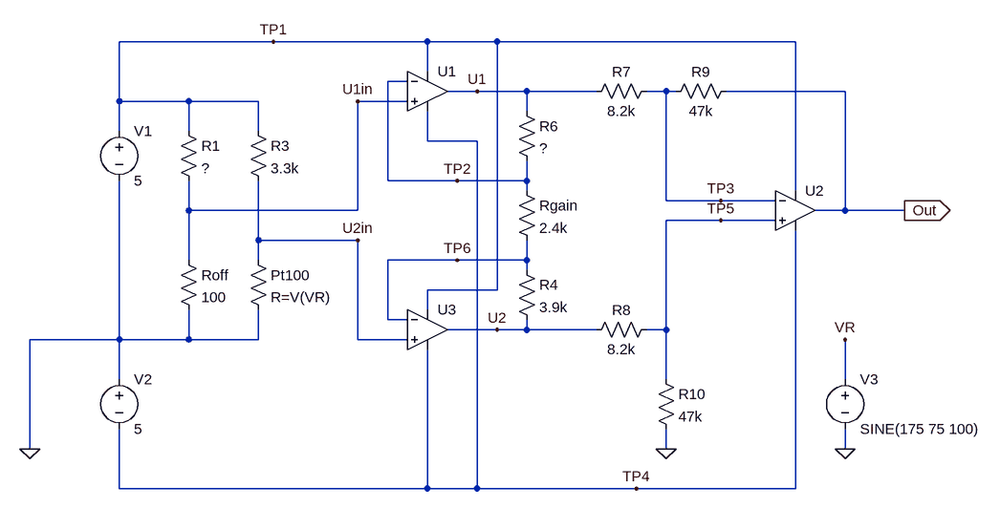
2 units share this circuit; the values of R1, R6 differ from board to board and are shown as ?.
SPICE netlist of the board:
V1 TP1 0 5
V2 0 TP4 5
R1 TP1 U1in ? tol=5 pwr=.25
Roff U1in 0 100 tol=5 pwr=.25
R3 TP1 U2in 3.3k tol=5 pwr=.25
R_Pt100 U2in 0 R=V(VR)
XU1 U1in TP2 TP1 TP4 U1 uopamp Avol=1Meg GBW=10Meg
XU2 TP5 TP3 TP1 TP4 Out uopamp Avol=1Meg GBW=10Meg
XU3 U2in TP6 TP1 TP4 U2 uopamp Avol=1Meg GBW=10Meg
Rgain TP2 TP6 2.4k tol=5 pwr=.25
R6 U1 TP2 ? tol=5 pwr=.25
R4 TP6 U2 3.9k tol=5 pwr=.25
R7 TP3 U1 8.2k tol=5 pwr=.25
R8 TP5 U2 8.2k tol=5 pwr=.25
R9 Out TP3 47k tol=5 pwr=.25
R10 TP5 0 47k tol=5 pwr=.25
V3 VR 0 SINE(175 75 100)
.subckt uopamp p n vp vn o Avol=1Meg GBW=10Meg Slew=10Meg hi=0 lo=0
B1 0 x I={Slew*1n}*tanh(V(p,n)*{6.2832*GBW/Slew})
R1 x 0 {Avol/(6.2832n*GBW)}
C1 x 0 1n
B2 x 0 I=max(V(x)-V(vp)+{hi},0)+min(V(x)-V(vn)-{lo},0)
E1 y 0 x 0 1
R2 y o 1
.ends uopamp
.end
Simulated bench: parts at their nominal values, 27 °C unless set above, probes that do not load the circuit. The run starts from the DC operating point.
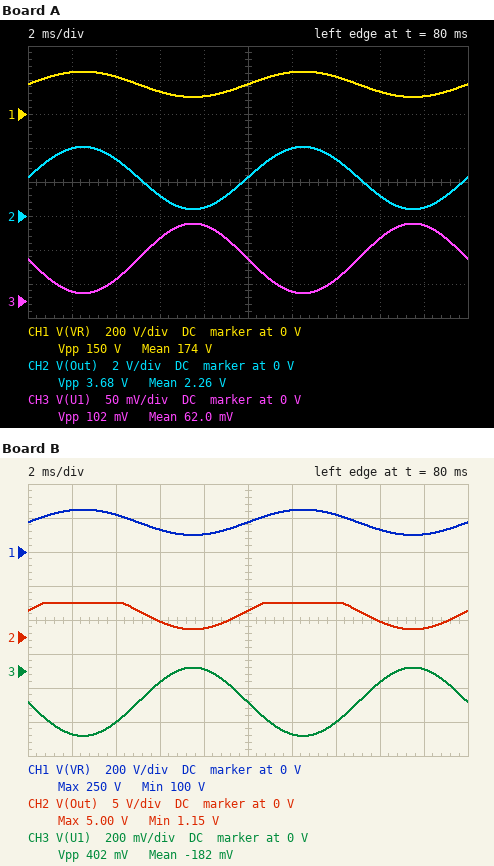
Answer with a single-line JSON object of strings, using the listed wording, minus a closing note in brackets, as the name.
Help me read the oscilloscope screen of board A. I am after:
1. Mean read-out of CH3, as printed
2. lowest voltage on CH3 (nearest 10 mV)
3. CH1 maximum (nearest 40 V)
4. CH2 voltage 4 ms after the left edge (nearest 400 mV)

{"Mean read-out of CH3, as printed": "62.0 mV", "lowest voltage on CH3": "10 mV", "CH1 maximum": "240 V", "CH2 voltage 4 ms after the left edge": "3.2 V"}
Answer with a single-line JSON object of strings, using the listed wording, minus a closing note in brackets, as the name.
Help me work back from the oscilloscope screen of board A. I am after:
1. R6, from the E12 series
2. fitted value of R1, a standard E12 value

{"R6, from the E12 series": "1.2 kΩ", "fitted value of R1, a standard E12 value": "3.9 kΩ"}
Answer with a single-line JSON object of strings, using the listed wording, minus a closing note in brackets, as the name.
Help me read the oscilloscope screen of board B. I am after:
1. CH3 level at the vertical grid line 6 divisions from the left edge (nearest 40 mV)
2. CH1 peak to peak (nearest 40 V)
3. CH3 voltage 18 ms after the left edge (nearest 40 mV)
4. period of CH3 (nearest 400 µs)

{"CH3 level at the vertical grid line 6 divisions from the left edge": "-360 mV", "CH1 peak to peak": "160 V", "CH3 voltage 18 ms after the left edge": "0 V", "period of CH3": "10.0 ms"}
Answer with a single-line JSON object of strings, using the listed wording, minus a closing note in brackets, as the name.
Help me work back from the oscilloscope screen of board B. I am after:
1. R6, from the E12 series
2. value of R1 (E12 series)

{"R6, from the E12 series": "4.7 kΩ", "value of R1": "4.7 kΩ"}
